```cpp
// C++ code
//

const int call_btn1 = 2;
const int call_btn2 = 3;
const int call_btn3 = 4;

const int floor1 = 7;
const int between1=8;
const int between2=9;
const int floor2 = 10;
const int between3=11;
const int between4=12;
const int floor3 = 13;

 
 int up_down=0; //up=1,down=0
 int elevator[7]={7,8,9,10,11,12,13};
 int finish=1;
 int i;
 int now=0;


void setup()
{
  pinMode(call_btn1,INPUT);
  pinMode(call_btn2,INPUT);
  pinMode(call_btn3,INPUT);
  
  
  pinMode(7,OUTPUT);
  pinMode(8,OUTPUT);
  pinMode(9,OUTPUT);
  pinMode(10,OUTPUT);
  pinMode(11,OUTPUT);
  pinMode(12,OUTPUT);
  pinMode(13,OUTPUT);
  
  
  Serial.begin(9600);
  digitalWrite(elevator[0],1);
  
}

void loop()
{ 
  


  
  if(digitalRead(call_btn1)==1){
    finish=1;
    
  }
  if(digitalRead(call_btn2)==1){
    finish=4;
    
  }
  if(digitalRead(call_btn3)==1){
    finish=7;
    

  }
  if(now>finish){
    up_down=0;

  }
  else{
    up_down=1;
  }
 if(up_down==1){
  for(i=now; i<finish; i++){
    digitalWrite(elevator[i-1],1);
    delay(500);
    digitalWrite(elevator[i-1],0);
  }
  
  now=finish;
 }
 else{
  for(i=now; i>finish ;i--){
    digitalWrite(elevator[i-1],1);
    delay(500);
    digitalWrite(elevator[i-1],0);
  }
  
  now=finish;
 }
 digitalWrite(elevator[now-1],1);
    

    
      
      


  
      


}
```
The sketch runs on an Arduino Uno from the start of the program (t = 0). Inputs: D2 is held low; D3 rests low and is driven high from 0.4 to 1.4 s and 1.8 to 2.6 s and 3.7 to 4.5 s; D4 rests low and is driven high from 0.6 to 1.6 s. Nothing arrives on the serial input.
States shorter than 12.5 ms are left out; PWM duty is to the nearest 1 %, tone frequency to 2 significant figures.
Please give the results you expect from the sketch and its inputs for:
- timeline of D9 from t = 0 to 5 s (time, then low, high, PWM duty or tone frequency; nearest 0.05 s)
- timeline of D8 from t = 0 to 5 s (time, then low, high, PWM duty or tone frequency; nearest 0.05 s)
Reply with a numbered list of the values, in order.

1. 0 s low; 1.5 s high; 2 s low
2. 0 s low; 1 s high; 1.5 s low
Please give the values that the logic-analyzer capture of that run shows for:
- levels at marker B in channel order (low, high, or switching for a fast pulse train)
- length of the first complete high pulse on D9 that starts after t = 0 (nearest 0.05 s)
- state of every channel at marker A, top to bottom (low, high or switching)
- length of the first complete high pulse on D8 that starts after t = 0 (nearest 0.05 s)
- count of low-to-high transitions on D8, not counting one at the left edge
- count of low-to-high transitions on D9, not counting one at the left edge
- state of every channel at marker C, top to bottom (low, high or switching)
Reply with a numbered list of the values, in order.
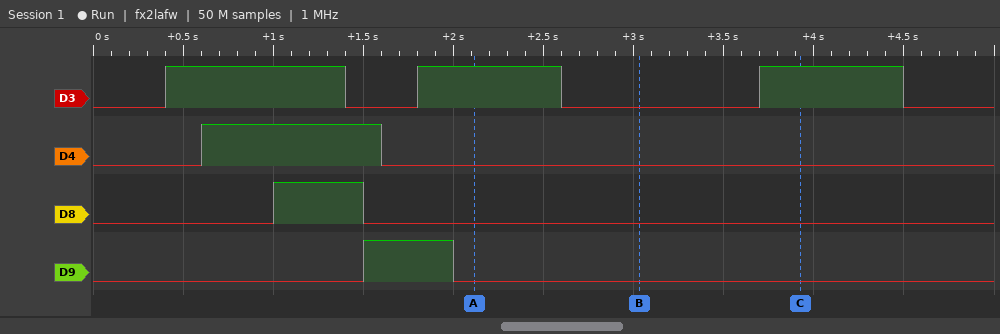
1. D3 low, D4 low, D8 low, D9 low
2. 0.50 s
3. D3 high, D4 low, D8 low, D9 low
4. 0.50 s
5. 1
6. 1
7. D3 high, D4 low, D8 low, D9 low
